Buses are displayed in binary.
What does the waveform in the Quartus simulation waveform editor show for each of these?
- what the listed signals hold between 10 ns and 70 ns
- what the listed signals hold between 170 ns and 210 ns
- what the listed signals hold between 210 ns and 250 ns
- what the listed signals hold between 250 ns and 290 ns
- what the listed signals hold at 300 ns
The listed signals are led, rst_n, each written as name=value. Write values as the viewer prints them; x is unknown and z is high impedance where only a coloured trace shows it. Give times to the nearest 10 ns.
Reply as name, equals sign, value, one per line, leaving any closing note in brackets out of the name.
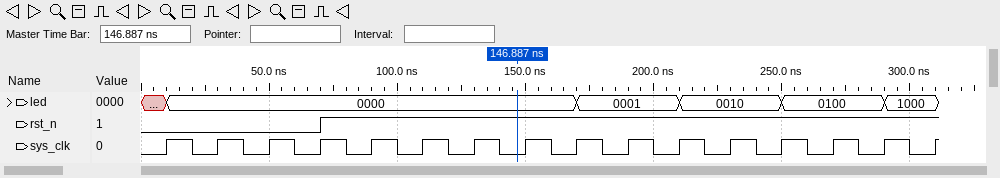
what the listed signals hold between 10 ns and 70 ns = led=0000, rst_n=0
what the listed signals hold between 170 ns and 210 ns = led=0001, rst_n=1
what the listed signals hold between 210 ns and 250 ns = led=0010, rst_n=1
what the listed signals hold between 250 ns and 290 ns = led=0100, rst_n=1
what the listed signals hold at 300 ns = led=1000, rst_n=1
